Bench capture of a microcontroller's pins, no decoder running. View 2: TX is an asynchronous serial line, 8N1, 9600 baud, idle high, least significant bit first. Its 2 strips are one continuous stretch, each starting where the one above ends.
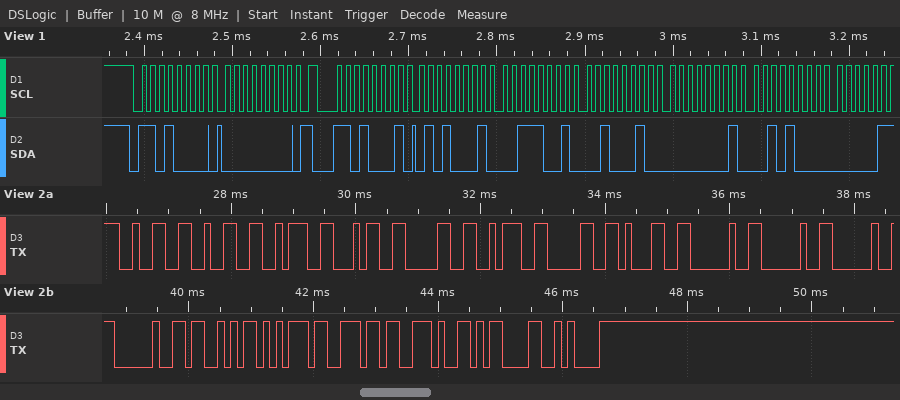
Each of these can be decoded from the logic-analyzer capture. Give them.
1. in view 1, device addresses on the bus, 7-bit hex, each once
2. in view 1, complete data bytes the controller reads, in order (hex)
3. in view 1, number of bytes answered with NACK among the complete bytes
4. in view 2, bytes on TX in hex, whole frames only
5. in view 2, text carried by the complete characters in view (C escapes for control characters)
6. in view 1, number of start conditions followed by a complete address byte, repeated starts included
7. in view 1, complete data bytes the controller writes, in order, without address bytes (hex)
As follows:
0x68
51 39 22 01 28
0
32 32 3A 34 30 3A 30 31 20 20 20 20 53 75 6E 2E 0D 0A
"22:40:01    Sun.\r\n"
2
00
